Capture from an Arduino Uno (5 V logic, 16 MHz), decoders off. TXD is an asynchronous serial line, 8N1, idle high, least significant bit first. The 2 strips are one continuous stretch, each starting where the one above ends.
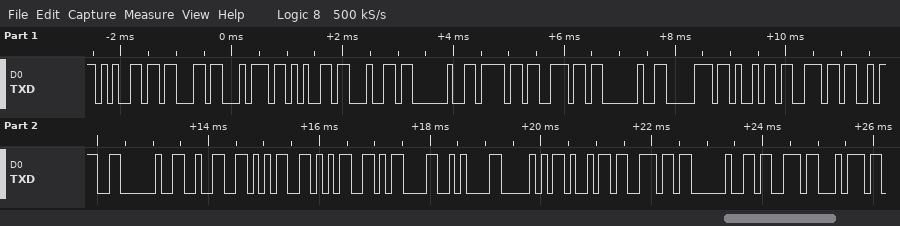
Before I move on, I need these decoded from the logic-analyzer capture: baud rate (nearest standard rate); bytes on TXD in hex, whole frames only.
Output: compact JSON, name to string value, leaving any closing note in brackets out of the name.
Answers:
{"baud rate": "9600 baud", "bytes on TXD in hex, whole frames only": "65 63 74 65 64 20 6F 6E 20 70 69 6E 3A 20 32 35 35 0D 0A 50 69 6E 20 73 74"}
